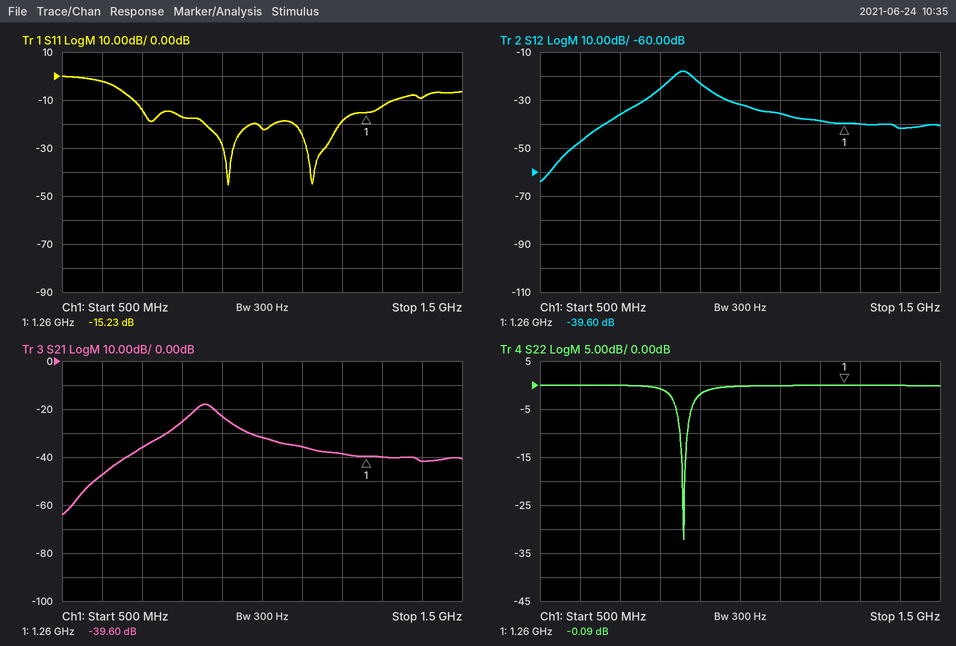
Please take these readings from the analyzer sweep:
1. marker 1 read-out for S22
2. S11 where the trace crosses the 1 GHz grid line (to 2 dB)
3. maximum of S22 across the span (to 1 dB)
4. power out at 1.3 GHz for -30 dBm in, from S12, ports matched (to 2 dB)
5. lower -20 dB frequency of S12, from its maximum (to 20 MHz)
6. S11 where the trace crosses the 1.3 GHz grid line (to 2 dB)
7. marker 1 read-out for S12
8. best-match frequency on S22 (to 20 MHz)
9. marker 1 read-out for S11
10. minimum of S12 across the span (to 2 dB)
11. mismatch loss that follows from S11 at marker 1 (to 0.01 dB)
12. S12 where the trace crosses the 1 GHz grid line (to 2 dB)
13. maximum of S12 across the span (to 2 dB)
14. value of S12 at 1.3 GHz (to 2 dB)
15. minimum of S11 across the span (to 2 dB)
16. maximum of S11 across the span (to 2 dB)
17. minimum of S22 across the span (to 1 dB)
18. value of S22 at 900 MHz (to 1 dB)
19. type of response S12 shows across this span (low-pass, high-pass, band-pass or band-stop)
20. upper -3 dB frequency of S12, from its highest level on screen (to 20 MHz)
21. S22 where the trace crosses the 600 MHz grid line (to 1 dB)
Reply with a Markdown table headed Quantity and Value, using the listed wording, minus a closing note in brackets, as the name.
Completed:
| Quantity | Value |
|---|---|
| marker 1 read-out for S22 | -0.09 dB |
| S11 where the trace crosses the 1 GHz grid line | -22 dB |
| maximum of S22 across the span | 0 dB |
| power out at 1.3 GHz for -30 dBm in, from S12, ports matched | -70 dBm |
| lower -20 dB frequency of S12, from its maximum | 680 MHz |
| S11 where the trace crosses the 1.3 GHz grid line | -12 dB |
| marker 1 read-out for S12 | -39.60 dB |
| best-match frequency on S22 | 860 MHz |
| marker 1 read-out for S11 | -15.23 dB |
| minimum of S12 across the span | -64 dB |
| mismatch loss that follows from S11 at marker 1 | 0.13 dB |
| S12 where the trace crosses the 1 GHz grid line | -32 dB |
| maximum of S12 across the span | -18 dB |
| value of S12 at 1.3 GHz | -40 dB |
| minimum of S11 across the span | -46 dB |
| maximum of S11 across the span | 0 dB |
| minimum of S22 across the span | -32 dB |
| value of S22 at 900 MHz | -2 dB |
| type of response S12 shows across this span | band-pass |
| upper -3 dB frequency of S12, from its highest level on screen | 880 MHz |
| S22 where the trace crosses the 600 MHz grid line | 0 dB |
